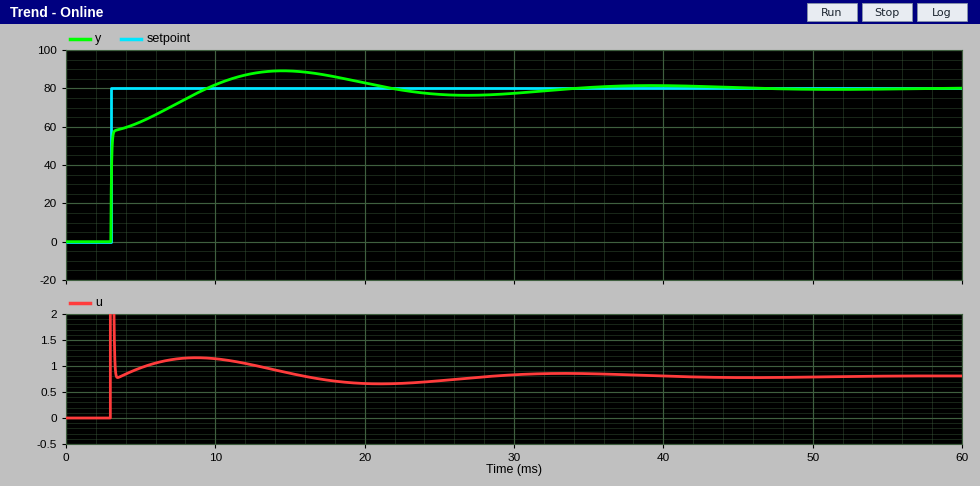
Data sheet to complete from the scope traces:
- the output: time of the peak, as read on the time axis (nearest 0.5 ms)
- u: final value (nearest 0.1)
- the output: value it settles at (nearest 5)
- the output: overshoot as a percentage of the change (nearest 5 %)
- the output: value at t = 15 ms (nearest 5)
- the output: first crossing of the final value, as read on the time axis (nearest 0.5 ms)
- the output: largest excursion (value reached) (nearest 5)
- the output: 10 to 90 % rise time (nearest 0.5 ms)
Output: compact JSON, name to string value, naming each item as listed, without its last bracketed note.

{"the output: time of the peak, as read on the time axis": "14.5 ms", "u: final value": "0.8", "the output: value it settles at": "80", "the output: overshoot as a percentage of the change": "10 %", "the output: value at t = 15 ms": "90", "the output: first crossing of the final value, as read on the time axis": "9.5 ms", "the output: largest excursion (value reached)": "90", "the output: 10 to 90 % rise time": "4.5 ms"}
